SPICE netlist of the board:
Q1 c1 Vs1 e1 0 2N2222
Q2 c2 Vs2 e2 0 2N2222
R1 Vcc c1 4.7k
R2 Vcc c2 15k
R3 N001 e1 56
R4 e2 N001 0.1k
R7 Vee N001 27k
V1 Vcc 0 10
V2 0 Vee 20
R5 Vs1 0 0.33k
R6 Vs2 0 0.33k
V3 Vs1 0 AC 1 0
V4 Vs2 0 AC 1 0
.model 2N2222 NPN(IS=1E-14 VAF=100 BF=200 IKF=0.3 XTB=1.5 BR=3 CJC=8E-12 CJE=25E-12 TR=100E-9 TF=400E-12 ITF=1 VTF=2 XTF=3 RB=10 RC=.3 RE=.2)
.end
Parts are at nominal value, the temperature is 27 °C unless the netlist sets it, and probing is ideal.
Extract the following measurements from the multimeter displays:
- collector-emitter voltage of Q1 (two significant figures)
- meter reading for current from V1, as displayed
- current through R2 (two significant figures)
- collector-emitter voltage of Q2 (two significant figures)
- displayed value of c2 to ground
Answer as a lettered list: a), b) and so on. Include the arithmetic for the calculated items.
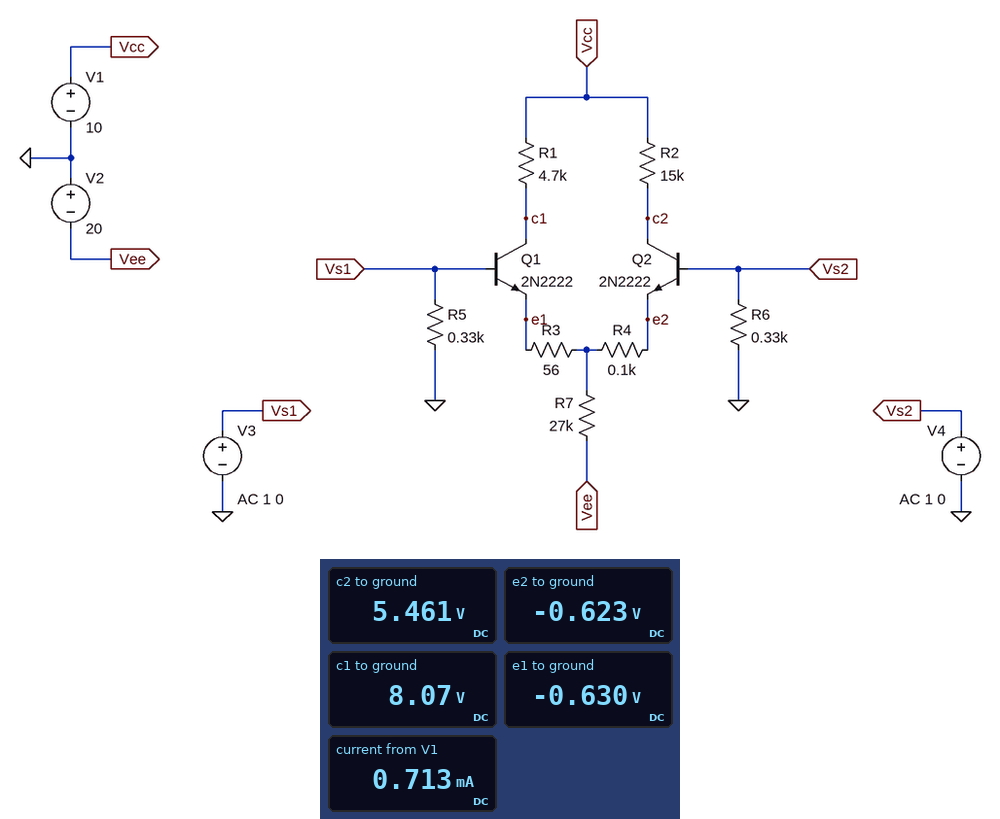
a) 8.07 V - (-630 mV) = 8.7 V
b) 0.713 mA
c) (10 V - 5.461 V) / 15 kΩ = 300 µA
d) 5.461 V - (-623 mV) = 6.1 V
e) 5.461 V
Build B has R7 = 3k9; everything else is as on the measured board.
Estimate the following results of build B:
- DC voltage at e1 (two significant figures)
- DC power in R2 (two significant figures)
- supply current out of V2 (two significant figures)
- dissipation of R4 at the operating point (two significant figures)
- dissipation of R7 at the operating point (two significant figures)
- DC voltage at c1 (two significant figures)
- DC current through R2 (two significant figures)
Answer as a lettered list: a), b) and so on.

a) -710 mV
b) 7.6 mW
c) 4.9 mA
d) 310 µW
e) 94 mW
f) -690 mV
g) 710 µA
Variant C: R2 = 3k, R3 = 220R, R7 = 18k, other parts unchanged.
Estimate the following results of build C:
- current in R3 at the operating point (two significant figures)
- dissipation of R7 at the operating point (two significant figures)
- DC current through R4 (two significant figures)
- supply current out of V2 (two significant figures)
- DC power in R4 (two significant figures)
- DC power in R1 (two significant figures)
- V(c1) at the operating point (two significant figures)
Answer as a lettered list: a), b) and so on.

a) 380 µA
b) 21 mW
c) 690 µA
d) 1.1 mA
e) 47 µW
f) 680 µW
g) 8.2 V
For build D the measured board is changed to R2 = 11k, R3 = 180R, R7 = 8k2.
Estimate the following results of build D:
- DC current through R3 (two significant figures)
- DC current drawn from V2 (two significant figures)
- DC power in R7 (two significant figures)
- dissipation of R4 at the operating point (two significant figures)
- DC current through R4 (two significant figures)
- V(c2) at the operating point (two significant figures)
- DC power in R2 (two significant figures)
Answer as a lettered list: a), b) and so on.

a) 950 µA
b) 2.3 mA
c) 45 mW
d) 190 µW
e) 1.4 mA
f) -660 mV
g) 10 mW
